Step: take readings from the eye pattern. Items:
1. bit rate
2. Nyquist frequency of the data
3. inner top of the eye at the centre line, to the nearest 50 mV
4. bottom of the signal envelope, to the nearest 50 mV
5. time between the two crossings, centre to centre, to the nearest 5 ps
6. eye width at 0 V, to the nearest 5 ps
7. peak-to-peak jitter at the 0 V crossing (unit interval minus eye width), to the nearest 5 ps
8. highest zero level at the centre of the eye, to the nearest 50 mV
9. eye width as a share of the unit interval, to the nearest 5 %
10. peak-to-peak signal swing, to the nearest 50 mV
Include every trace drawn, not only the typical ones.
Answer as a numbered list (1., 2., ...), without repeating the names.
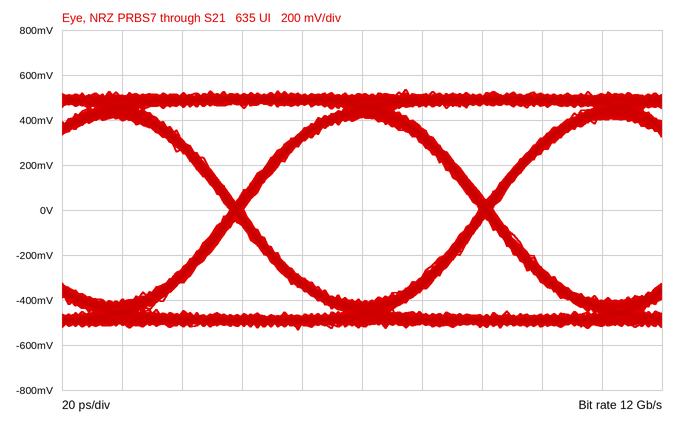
1. 12 Gb/s
2. 6 GHz
3. 400 mV
4. -550 mV
5. 85 ps
6. 80 ps
7. 5 ps
8. -400 mV
9. 95 %
10. 1.05 V
